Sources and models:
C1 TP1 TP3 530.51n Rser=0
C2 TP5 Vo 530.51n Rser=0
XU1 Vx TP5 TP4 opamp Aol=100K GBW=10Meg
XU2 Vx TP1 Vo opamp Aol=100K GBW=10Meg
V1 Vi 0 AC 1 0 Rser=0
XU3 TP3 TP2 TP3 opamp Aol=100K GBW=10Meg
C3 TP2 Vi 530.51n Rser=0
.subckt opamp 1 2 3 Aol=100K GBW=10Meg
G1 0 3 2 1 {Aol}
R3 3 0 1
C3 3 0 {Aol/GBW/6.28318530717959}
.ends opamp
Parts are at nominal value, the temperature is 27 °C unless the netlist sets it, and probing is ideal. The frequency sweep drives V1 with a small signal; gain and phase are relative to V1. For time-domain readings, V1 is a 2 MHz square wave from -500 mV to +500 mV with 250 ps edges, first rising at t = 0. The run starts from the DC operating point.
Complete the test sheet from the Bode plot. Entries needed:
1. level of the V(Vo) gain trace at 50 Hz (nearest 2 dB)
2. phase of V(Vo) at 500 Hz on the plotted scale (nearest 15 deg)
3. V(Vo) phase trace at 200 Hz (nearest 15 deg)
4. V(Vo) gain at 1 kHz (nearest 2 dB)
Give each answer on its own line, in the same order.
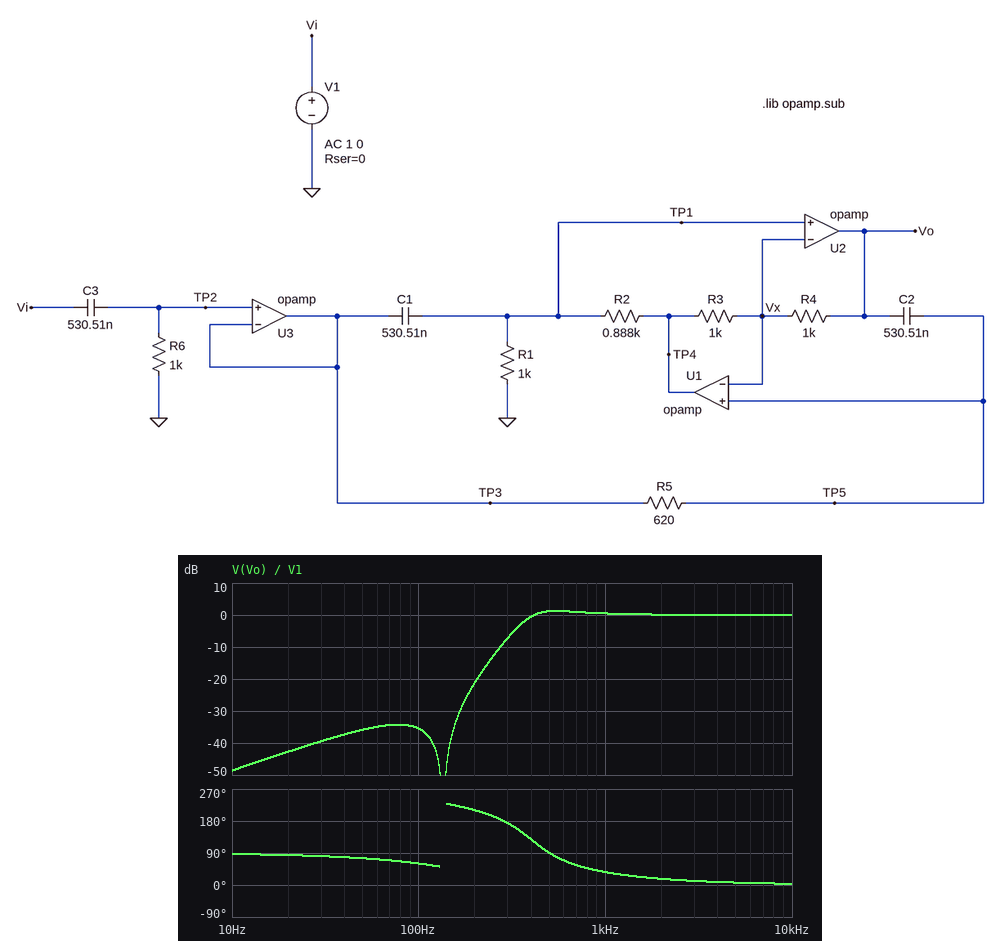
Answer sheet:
-36 dB
90 deg
210 deg
0 dB
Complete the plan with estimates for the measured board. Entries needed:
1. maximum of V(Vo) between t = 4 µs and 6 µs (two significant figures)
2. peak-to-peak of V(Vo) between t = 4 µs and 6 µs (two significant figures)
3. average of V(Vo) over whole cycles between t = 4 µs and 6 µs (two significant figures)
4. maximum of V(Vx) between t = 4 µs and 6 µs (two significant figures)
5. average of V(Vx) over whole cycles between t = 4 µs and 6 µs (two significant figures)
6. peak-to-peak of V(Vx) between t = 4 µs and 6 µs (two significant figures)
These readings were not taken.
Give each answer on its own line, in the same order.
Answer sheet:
1.1 V
1.3 V
490 mV
1.0 V
490 mV
1.1 V
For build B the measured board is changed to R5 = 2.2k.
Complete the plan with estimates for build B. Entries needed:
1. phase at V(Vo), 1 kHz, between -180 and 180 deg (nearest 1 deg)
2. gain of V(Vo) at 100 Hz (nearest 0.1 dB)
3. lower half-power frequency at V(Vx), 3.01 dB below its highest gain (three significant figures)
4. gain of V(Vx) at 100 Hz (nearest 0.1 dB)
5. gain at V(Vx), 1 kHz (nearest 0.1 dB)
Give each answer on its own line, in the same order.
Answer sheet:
34 deg
-29.7 dB
516 Hz
-12.3 dB
-0.8 dB
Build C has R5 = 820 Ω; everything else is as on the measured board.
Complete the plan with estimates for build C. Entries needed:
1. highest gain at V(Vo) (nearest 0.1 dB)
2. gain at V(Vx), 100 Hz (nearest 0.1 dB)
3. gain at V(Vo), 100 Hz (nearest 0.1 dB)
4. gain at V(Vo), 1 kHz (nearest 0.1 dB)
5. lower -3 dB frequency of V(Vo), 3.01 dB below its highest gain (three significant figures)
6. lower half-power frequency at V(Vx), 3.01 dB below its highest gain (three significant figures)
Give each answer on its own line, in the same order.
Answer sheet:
0.4 dB
-10.3 dB
-39.7 dB
0.2 dB
338 Hz
596 Hz
